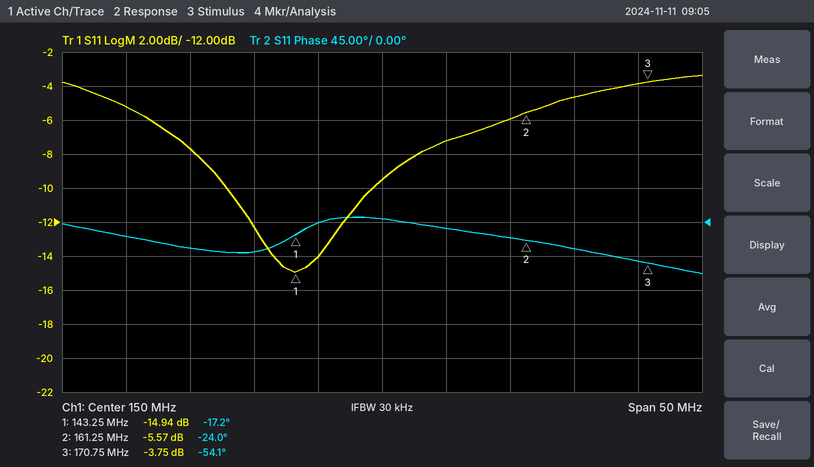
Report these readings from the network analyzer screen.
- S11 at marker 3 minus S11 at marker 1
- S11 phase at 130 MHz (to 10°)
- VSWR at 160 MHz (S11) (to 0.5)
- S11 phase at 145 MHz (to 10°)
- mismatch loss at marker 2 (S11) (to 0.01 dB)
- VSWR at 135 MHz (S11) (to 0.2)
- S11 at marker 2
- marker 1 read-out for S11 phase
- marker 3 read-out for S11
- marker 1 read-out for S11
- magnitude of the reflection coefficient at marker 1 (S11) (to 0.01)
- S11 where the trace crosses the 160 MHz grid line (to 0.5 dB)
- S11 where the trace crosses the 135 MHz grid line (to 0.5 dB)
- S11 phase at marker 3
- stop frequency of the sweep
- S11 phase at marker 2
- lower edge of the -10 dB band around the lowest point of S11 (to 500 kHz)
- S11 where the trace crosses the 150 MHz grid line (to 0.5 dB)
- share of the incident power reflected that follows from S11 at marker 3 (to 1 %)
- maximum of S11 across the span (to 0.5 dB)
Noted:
11.19 dB
-20°
3.0
0°
1.41 dB
2.4
-5.57 dB
-17.2°
-3.75 dB
-14.94 dB
0.18
-6.0 dB
-7.5 dB
-54.1°
175 MHz
-24.0°
138.0 MHz
-9.5 dB
42 %
-3.5 dB
